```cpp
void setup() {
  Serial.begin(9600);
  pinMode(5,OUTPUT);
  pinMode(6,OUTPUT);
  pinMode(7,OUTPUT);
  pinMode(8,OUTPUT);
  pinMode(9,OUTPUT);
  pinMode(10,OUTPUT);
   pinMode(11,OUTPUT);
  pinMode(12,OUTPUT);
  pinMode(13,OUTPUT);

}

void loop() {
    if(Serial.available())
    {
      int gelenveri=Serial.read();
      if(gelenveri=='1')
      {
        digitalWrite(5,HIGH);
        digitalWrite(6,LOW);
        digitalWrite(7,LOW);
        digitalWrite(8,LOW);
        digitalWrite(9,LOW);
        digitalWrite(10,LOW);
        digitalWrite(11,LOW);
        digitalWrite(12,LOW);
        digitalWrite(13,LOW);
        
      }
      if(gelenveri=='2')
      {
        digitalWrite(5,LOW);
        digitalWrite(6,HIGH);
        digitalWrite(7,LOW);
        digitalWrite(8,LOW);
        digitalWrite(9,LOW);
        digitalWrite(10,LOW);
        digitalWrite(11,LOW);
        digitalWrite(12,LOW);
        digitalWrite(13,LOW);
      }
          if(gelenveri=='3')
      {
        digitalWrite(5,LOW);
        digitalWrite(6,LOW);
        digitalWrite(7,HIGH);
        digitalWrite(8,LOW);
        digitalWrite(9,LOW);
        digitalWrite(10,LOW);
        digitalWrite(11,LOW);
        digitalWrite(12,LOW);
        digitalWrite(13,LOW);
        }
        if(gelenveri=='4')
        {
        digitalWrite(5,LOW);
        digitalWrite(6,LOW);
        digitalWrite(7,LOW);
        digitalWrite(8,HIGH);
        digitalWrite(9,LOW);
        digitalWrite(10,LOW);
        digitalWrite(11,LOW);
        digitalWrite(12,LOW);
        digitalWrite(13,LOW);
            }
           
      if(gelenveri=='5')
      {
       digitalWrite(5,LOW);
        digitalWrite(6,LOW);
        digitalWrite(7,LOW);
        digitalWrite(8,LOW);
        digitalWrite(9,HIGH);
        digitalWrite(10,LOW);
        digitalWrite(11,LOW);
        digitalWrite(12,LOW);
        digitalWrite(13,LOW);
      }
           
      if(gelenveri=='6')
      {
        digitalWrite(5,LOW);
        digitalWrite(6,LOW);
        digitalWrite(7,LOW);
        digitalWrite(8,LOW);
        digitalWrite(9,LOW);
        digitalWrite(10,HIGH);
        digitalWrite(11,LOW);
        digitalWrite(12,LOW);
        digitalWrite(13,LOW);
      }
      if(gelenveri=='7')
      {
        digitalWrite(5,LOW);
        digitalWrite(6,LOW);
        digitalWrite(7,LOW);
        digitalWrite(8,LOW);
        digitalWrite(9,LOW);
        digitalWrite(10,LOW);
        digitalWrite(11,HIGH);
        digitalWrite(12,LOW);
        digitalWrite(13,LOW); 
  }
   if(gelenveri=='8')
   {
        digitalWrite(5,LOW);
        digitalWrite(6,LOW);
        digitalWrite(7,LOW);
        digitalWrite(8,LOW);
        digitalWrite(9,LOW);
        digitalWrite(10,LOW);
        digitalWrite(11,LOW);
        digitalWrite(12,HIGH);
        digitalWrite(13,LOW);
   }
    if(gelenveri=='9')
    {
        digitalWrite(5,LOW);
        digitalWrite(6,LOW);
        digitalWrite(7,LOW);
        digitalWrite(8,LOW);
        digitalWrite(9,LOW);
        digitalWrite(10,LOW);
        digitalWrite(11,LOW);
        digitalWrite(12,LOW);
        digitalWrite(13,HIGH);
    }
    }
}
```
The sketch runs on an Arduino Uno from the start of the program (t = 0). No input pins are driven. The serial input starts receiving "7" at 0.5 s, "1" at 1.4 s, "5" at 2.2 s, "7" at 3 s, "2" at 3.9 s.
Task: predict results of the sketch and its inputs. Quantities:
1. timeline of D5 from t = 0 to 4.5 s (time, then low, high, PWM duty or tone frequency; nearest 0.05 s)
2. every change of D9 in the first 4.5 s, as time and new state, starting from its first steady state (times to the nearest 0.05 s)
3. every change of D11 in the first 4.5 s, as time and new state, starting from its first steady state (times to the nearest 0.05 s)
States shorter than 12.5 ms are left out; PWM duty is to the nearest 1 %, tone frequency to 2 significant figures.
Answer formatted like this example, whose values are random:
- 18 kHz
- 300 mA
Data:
- 0 s low; 1.4 s high; 2.2 s low
- 0 s low; 2.2 s high; 3 s low
- 0 s low; 0.5 s high; 1.4 s low; 3 s high; 3.9 s low
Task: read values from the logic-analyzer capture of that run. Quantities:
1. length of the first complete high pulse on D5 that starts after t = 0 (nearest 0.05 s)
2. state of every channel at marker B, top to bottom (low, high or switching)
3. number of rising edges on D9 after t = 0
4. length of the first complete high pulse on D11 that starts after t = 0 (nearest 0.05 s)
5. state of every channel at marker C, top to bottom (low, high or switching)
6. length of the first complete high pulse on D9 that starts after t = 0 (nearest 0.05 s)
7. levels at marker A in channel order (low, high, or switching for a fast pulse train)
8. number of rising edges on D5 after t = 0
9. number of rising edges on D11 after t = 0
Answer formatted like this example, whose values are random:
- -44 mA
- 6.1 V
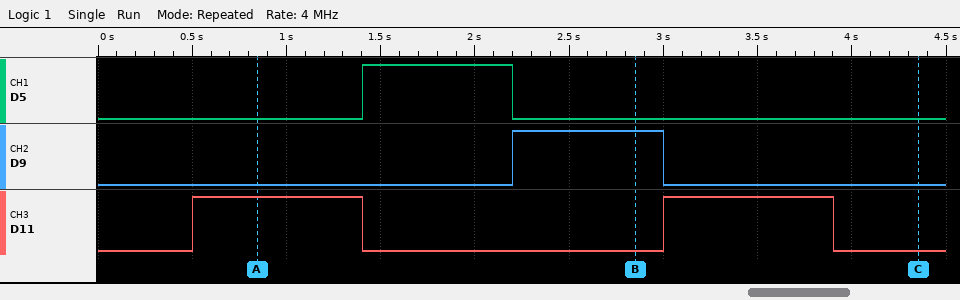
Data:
- 0.80 s
- D5 low, D9 high, D11 low
- 1
- 0.90 s
- D5 low, D9 low, D11 low
- 0.80 s
- D5 low, D9 low, D11 high
- 1
- 2
